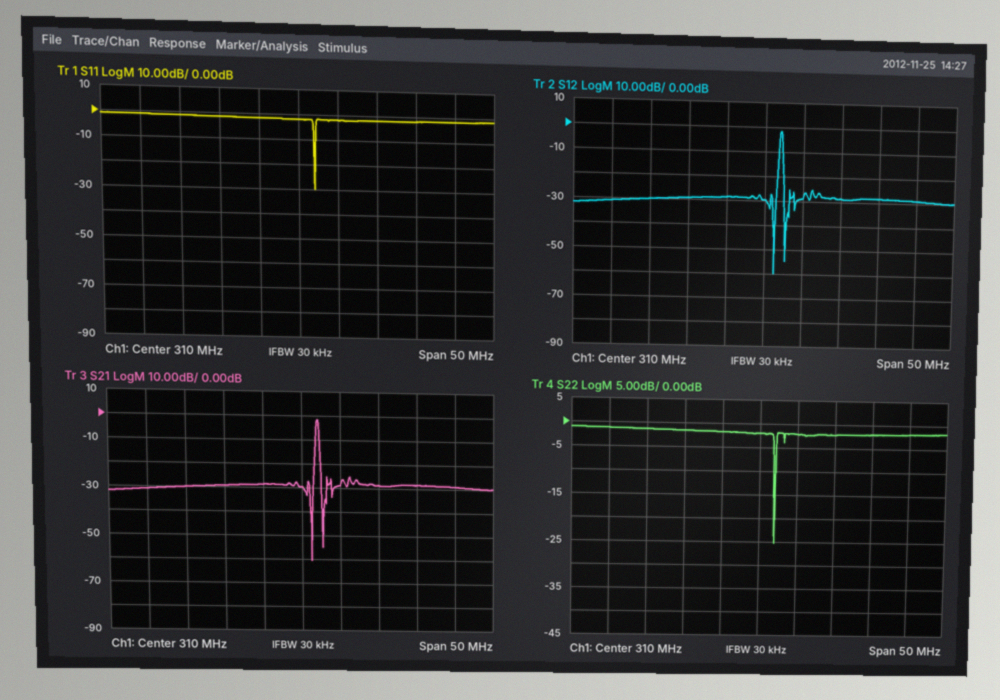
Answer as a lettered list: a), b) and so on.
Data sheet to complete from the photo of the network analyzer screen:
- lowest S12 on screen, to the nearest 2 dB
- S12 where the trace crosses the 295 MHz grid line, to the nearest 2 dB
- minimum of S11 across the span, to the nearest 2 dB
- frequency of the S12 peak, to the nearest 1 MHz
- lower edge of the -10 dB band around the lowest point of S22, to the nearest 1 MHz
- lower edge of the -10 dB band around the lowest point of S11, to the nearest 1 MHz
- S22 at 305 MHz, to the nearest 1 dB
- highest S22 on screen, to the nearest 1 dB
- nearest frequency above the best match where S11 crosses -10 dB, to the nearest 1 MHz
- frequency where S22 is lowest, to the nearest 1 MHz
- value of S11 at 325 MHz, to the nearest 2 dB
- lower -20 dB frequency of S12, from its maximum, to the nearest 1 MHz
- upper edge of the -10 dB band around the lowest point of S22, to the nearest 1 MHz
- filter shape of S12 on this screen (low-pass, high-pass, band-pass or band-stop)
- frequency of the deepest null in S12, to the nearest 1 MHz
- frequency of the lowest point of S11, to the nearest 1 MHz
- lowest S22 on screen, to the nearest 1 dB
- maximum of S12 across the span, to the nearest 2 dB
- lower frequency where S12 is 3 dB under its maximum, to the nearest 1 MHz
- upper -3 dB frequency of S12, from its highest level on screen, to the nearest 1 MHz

a) -60 dB
b) -30 dB
c) -30 dB
d) 312 MHz
e) 312 MHz
f) 312 MHz
g) -2 dB
h) -1 dB
i) 312 MHz
j) 312 MHz
k) -2 dB
l) 312 MHz
m) 312 MHz
n) band-pass
o) 311 MHz
p) 312 MHz
q) -25 dB
r) -2 dB
s) 312 MHz
t) 312 MHz
